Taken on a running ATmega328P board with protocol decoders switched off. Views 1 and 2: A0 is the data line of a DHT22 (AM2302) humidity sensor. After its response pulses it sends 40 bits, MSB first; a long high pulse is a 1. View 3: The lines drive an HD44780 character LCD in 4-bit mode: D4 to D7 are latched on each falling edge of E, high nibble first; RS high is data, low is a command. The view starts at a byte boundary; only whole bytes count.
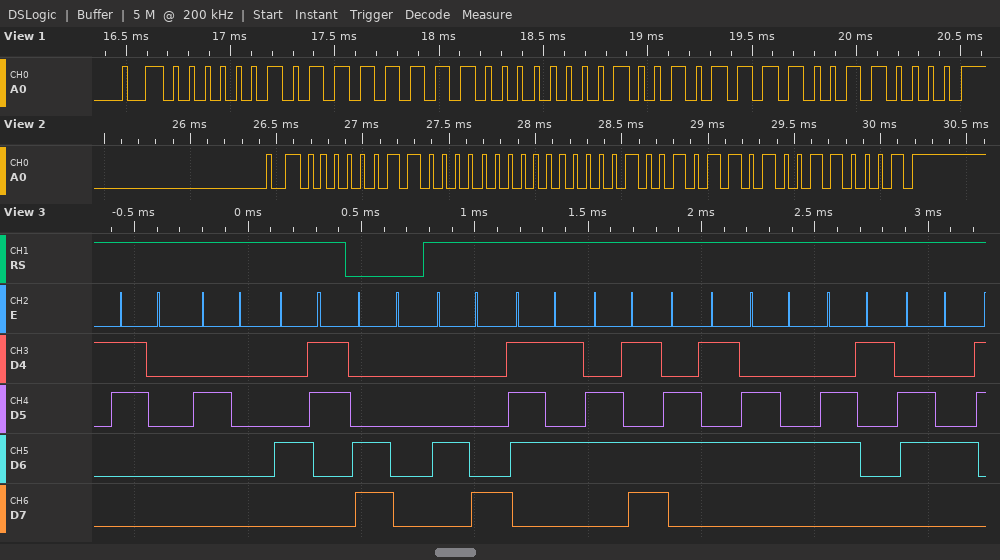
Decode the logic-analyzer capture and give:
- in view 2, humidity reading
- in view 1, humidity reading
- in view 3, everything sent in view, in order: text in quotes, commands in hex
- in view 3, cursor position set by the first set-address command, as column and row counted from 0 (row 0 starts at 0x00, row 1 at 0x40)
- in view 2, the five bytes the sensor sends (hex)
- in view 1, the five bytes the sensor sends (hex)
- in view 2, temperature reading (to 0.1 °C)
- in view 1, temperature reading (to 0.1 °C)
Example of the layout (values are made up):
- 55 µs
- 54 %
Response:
- 76.8 %
- 76.6 %
- "0 C" 0xC0 "Humedad"
- column 0, row 1
- 03 00 01 2D 31
- 02 FE 01 2F 30
- 30.1 °C
- 30.3 °C
